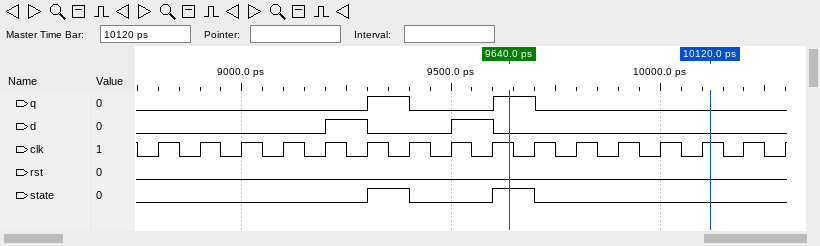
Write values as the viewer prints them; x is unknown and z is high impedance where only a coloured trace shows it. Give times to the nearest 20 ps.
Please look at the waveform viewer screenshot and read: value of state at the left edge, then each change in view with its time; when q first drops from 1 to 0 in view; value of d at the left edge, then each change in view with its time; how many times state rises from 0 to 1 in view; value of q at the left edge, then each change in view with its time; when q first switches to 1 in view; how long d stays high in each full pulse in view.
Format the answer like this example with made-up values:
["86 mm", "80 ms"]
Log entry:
["0, 1 at 9300 ps, 0 at 9400 ps, 1 at 9600 ps, 0 at 9700 ps", "9400 ps", "0, 1 at 9200 ps, 0 at 9300 ps, 1 at 9500 ps, 0 at 9600 ps", "2", "0, 1 at 9300 ps, 0 at 9400 ps, 1 at 9600 ps, 0 at 9700 ps", "9300 ps", "100 ps, 100 ps"]
